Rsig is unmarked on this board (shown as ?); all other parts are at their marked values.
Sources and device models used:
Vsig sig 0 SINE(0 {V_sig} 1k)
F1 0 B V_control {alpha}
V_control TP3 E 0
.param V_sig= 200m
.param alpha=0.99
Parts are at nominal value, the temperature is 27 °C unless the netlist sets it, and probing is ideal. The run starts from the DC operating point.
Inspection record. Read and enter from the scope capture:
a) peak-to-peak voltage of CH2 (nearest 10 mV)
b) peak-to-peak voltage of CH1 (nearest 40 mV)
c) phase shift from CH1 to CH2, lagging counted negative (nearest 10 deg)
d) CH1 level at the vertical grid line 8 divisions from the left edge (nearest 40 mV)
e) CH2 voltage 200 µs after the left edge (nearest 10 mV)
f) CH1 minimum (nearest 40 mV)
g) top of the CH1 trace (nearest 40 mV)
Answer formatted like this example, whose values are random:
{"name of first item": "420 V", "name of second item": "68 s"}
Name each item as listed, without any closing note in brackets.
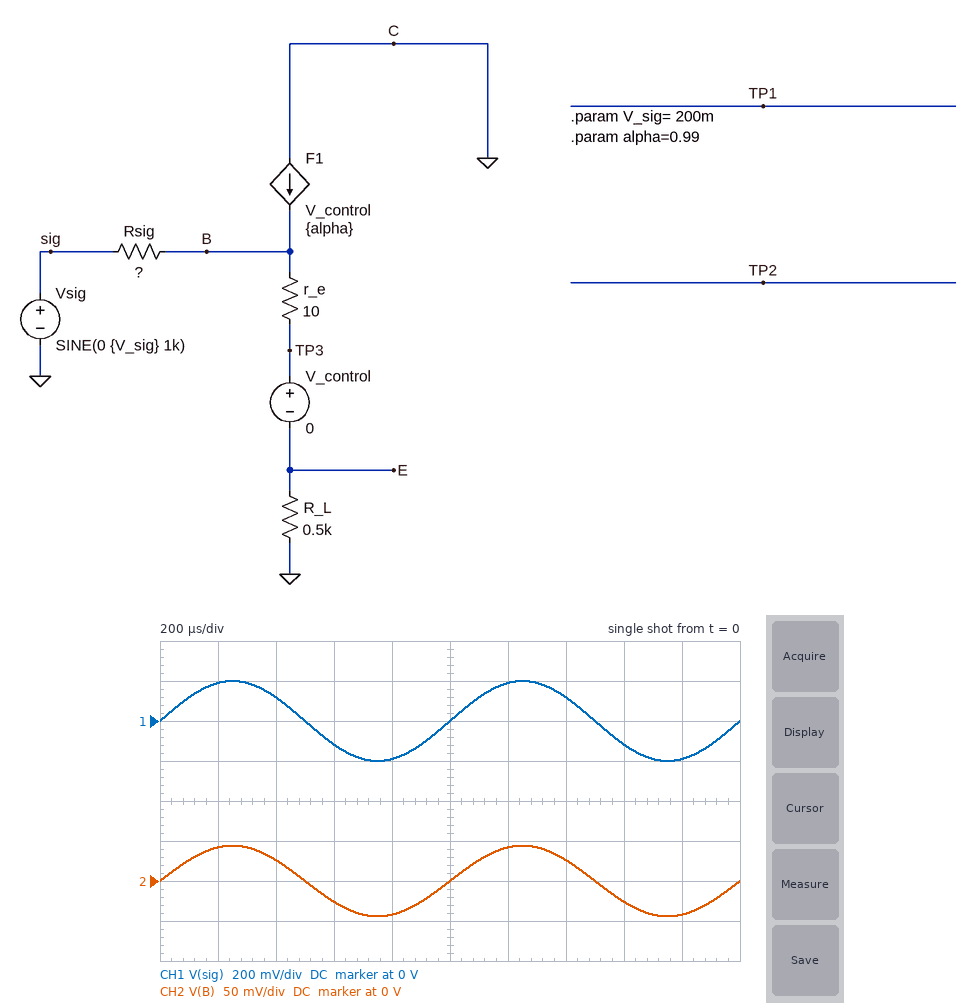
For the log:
{"peak-to-peak voltage of CH2": "90 mV", "peak-to-peak voltage of CH1": "400 mV", "phase shift from CH1 to CH2, lagging counted negative": "0 deg", "CH1 level at the vertical grid line 8 divisions from the left edge": "-120 mV", "CH2 voltage 200 µs after the left edge": "40 mV", "CH1 minimum": "-200 mV", "top of the CH1 trace": "200 mV"}
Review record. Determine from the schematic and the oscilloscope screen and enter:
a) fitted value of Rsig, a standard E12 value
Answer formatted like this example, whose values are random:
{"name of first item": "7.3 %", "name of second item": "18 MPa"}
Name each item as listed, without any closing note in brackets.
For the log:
{"fitted value of Rsig, a standard E12 value": "180 kΩ"}
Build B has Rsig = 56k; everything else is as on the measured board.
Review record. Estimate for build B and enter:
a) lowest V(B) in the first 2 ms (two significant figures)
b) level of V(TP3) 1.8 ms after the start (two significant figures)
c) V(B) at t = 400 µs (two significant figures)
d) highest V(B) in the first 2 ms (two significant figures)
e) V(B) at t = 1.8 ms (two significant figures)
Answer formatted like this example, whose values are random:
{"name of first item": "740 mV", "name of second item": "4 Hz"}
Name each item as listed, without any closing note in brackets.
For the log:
{"lowest V(B) in the first 2 ms": "-95 mV", "level of V(TP3) 1.8 ms after the start": "-89 mV", "V(B) at t = 400 µs": "56 mV", "highest V(B) in the first 2 ms": "95 mV", "V(B) at t = 1.8 ms": "-91 mV"}
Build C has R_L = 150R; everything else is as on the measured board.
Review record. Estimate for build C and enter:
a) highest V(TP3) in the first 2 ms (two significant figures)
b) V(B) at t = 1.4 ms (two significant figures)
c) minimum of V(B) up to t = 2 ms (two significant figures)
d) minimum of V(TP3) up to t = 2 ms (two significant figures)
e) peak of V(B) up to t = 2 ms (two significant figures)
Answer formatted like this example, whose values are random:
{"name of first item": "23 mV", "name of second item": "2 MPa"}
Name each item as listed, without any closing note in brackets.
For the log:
{"highest V(TP3) in the first 2 ms": "15 mV", "V(B) at t = 1.4 ms": "9.6 mV", "minimum of V(B) up to t = 2 ms": "-16 mV", "minimum of V(TP3) up to t = 2 ms": "-15 mV", "peak of V(B) up to t = 2 ms": "16 mV"}
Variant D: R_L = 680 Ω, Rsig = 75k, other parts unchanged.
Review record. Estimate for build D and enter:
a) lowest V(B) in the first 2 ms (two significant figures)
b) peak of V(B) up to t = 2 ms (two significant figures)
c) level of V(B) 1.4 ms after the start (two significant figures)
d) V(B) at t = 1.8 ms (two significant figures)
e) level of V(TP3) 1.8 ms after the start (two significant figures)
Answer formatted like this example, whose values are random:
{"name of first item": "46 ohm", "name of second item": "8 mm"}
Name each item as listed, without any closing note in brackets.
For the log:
{"lowest V(B) in the first 2 ms": "-96 mV", "peak of V(B) up to t = 2 ms": "96 mV", "level of V(B) 1.4 ms after the start": "56 mV", "V(B) at t = 1.8 ms": "-91 mV", "level of V(TP3) 1.8 ms after the start": "-90 mV"}
